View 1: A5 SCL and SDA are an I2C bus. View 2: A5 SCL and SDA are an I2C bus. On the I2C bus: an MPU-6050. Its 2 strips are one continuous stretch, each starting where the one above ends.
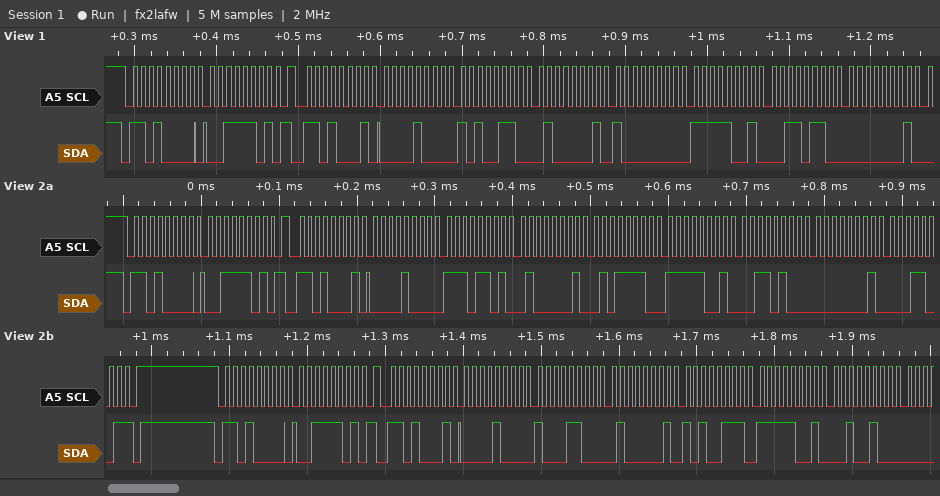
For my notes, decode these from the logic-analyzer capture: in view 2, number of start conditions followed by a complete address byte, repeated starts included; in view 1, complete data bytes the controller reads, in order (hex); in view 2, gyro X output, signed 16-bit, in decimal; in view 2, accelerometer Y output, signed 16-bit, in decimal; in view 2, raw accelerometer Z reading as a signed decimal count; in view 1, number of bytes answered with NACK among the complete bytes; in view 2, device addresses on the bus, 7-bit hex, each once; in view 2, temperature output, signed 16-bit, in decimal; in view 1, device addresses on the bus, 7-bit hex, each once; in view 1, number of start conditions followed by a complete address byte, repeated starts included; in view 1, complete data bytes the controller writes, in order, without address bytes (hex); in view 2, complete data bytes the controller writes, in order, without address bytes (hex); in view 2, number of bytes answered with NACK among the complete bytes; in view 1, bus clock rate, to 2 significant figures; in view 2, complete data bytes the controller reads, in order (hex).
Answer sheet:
4
08 A6 41 80 F9 36 01
281
2285
16734
0
0x68
-1740
0x68
2
3D
3D 3D
1
100 kHz
08 ED 41 5E F9 34 01 19 08 8C 41 A7 F9 24
